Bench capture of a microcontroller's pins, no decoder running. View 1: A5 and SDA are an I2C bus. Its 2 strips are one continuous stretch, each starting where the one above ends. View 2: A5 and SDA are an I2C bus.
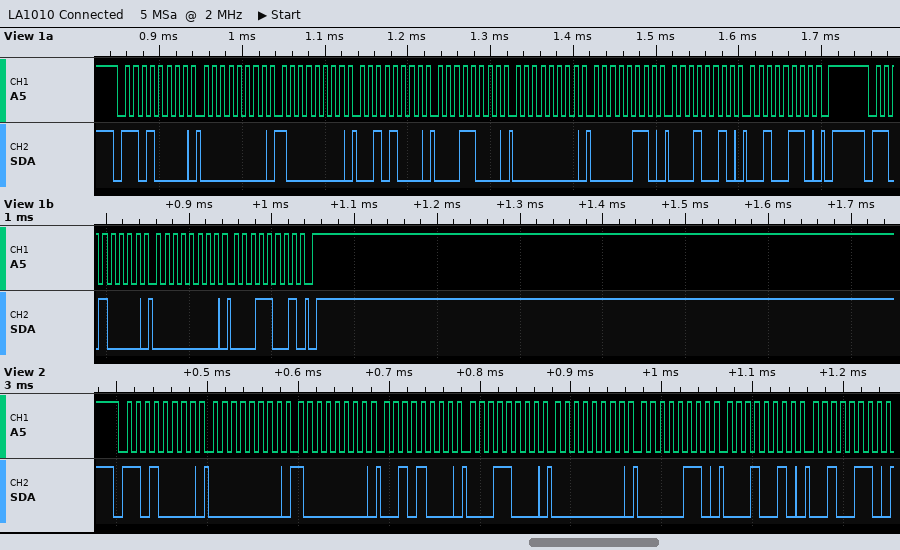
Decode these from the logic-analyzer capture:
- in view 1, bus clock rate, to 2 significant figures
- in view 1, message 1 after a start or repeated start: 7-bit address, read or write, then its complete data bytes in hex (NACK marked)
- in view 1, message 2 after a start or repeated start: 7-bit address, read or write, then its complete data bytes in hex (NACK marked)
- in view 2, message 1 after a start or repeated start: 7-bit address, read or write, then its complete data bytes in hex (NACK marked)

100 kHz
0x68 write: 00 80 28 18 00 06 12 26
0x68 write: 00 19
0x68 write: 00 80 28 18 00 06 12 26
